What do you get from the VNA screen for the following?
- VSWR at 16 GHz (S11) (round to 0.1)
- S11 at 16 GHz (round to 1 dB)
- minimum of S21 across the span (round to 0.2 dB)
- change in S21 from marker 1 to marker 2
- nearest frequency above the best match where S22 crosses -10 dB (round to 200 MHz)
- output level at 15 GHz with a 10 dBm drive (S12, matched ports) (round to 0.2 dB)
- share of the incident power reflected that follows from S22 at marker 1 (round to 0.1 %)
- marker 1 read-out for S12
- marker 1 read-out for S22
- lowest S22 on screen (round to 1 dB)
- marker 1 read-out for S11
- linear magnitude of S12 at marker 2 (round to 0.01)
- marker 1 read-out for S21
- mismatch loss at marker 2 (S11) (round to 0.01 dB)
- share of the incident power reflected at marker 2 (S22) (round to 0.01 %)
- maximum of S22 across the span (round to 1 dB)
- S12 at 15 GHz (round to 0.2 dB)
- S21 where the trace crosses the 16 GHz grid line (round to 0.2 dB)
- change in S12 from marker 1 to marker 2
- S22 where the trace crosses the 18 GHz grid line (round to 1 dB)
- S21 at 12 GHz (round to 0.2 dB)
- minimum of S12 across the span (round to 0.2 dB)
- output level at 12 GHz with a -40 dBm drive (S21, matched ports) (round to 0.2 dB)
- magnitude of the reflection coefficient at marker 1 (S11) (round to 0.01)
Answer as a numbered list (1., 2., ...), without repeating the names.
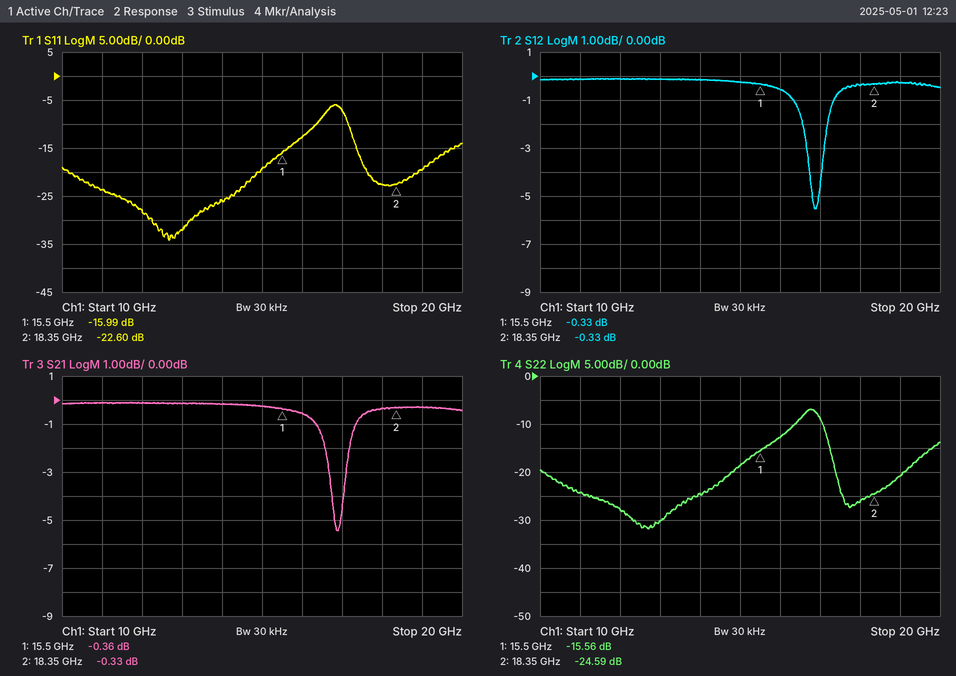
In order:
1. 1.6
2. -13 dB
3. -5.4 dB
4. 0.03 dB
5. 16.4 GHz
6. 9.8 dBm
7. 2.8 %
8. -0.33 dB
9. -15.56 dB
10. -32 dB
11. -15.99 dB
12. 0.96
13. -0.36 dB
14. 0.02 dB
15. 0.35 %
16. -7 dB
17. -0.2 dB
18. -0.6 dB
19. 0.00 dB
20. -26 dB
21. -0.2 dB
22. -5.6 dB
23. -40.2 dBm
24. 0.16
